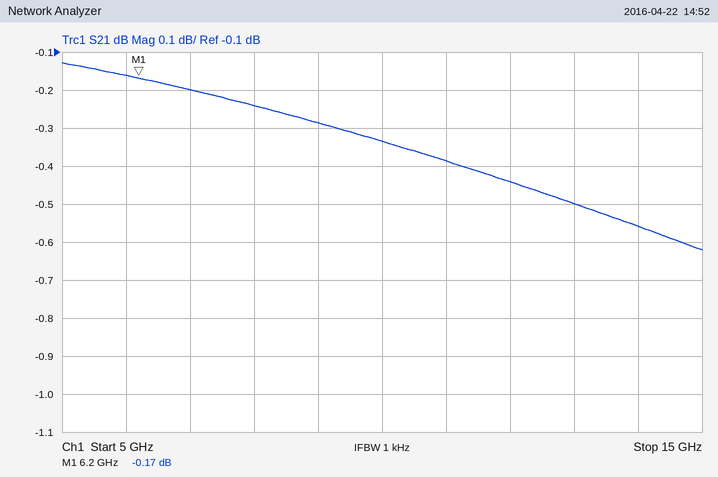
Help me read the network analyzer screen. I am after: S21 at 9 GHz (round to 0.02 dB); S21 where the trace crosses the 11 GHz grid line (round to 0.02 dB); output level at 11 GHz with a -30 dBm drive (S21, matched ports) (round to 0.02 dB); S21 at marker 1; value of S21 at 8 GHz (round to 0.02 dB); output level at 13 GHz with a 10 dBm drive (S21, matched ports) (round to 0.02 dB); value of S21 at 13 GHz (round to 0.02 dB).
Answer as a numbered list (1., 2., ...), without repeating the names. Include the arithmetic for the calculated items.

1. -0.28 dB
2. -0.38 dB
3. -30 dBm + (-0.38 dB) = -30.38 dBm
4. -0.17 dB
5. -0.24 dB
6. 10 dBm + (-0.50 dB) = 9.50 dBm
7. -0.50 dB
